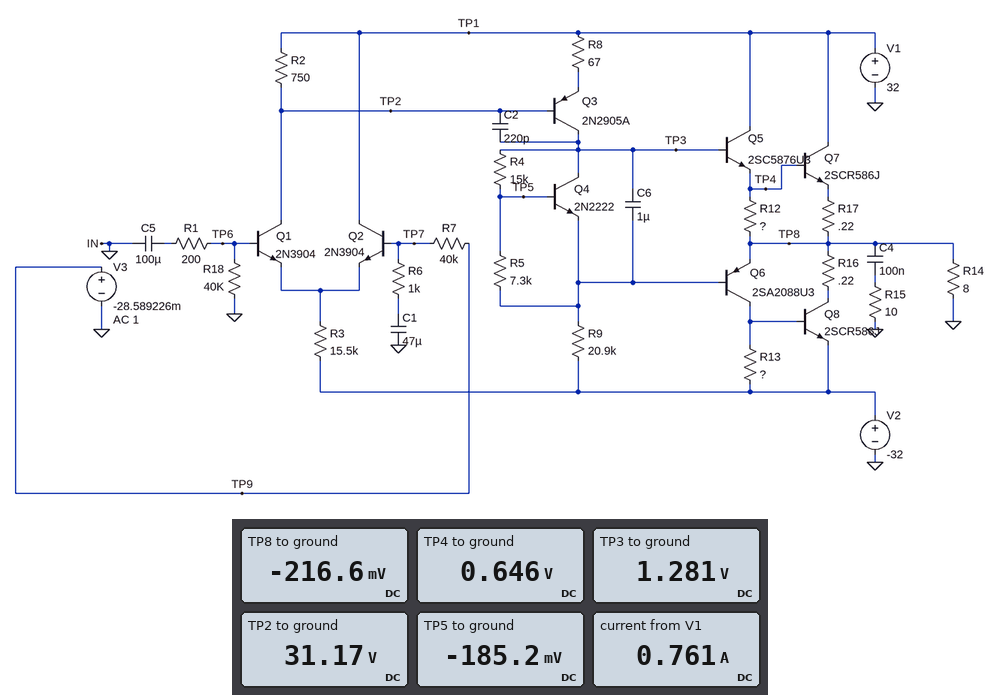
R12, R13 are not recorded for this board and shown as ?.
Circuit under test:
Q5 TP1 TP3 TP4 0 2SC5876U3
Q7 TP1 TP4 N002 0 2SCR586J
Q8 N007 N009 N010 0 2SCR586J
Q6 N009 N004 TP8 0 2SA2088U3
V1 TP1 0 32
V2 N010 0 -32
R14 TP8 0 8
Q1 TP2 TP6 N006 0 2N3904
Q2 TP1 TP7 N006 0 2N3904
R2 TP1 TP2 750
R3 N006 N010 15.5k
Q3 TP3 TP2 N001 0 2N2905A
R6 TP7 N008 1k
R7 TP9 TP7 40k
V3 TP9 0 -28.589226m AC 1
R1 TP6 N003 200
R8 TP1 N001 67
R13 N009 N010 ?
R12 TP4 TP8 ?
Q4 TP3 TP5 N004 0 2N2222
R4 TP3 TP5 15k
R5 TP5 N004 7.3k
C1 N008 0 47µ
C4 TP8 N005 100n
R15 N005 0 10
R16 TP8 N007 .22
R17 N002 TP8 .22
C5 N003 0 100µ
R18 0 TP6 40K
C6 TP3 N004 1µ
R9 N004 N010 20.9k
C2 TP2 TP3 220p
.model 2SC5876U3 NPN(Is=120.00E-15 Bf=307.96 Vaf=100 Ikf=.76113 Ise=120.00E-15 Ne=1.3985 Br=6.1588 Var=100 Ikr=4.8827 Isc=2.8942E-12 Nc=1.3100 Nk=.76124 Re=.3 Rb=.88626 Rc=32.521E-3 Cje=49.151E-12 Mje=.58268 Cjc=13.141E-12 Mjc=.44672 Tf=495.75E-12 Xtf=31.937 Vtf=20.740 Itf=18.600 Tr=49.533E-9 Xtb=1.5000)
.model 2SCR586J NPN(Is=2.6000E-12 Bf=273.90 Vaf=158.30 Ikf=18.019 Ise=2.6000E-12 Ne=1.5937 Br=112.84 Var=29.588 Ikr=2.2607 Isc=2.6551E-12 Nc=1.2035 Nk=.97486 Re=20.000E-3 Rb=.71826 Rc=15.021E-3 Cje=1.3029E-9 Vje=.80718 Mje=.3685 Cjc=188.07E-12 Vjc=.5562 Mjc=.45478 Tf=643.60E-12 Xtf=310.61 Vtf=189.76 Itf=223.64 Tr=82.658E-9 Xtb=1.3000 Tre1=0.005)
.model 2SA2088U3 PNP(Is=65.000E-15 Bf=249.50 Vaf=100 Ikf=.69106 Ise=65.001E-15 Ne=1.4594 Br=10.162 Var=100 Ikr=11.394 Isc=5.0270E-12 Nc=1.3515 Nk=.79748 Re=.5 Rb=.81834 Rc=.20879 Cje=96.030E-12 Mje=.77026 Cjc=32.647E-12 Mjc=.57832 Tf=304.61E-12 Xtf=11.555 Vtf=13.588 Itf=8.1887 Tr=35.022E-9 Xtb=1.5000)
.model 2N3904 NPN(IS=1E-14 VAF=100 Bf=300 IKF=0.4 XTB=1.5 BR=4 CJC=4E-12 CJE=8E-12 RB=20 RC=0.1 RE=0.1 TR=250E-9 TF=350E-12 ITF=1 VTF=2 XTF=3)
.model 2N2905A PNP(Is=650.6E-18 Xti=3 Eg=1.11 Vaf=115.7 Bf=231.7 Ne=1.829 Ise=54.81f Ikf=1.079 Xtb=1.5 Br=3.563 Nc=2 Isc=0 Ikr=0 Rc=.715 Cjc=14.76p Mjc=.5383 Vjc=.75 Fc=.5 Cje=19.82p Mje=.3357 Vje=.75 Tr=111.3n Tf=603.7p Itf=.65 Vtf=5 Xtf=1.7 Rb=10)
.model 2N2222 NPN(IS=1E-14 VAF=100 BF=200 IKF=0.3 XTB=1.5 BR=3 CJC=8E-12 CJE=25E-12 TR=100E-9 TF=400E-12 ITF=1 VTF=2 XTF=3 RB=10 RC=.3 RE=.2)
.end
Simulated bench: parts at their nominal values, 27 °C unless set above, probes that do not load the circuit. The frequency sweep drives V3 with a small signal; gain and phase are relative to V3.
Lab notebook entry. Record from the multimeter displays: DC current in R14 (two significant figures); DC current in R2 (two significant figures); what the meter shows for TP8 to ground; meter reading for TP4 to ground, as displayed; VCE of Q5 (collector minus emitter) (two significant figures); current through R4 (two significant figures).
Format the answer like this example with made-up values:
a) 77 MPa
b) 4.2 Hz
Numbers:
a) 27 mA
b) 1.1 mA
c) -216.6 mV
d) 0.646 V
e) 31 V
f) 98 µA
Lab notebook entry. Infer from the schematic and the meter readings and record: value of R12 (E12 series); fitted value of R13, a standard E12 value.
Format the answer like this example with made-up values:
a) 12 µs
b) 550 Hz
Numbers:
a) 220 Ω
b) 1.2 kΩ
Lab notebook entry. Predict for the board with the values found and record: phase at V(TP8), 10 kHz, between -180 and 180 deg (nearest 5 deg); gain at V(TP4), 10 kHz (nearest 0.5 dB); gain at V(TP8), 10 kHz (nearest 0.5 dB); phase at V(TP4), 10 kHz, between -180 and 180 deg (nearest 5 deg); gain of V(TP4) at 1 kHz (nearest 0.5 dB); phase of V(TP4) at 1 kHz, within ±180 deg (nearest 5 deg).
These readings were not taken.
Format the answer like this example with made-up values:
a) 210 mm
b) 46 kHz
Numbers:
a) 110 deg
b) 28.5 dB
c) 28.5 dB
d) 110 deg
e) 37.0 dB
f) 165 deg
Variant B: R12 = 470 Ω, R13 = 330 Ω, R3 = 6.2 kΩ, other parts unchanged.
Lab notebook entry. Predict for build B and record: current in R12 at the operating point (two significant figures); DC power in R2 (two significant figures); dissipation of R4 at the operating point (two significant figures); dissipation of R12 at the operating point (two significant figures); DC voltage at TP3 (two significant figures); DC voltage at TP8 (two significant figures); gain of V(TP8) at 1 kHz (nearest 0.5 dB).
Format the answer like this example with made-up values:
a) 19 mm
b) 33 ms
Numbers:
a) 3.5 mA
b) 1.5 mW
c) 170 µW
d) 5.7 mW
e) 32 V
f) 29 V
g) -26.0 dB
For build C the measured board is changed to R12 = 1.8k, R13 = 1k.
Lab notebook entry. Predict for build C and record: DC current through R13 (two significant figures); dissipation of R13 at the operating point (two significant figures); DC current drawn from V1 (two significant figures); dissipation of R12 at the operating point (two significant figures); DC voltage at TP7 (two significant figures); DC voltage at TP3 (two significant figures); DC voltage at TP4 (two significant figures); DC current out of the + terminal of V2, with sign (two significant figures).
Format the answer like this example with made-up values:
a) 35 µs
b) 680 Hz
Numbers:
a) 700 µA
b) 490 µW
c) 820 mA
d) 430 µW
e) -120 mV
f) 1.5 V
g) 880 mV
h) -820 mA
